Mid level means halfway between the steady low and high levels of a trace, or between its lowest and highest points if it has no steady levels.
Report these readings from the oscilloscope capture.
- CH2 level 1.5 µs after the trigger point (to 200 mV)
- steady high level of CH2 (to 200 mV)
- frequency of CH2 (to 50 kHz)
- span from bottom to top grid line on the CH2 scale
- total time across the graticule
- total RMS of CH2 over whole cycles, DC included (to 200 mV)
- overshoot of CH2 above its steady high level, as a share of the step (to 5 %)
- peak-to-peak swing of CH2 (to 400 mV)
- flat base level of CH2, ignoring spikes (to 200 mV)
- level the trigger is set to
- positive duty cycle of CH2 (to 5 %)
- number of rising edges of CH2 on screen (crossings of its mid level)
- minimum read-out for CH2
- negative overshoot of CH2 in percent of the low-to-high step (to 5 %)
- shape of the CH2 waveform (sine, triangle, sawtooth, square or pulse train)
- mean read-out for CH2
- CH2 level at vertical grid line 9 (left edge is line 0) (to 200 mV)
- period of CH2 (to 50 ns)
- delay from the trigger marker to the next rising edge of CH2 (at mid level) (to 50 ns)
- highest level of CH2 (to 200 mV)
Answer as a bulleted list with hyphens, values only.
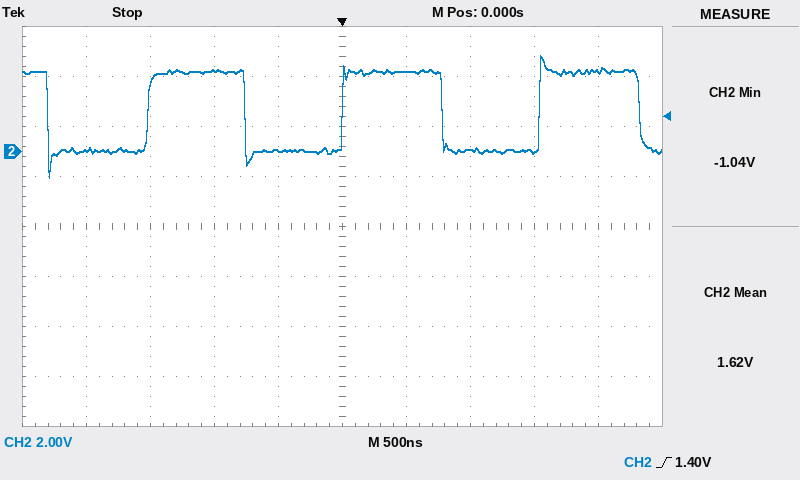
- 0.0 V
- 3.2 V
- 650 kHz
- 16 V
- 5 µs
- 2.2 V
- 20 %
- 4.8 V
- 0.0 V
- 1.40 V
- 50 %
- 3
- -1.04 V
- 35 %
- square
- 1.62 V
- 3.2 V
- 1.55 µs
- 1.55 µs
- 3.8 V
